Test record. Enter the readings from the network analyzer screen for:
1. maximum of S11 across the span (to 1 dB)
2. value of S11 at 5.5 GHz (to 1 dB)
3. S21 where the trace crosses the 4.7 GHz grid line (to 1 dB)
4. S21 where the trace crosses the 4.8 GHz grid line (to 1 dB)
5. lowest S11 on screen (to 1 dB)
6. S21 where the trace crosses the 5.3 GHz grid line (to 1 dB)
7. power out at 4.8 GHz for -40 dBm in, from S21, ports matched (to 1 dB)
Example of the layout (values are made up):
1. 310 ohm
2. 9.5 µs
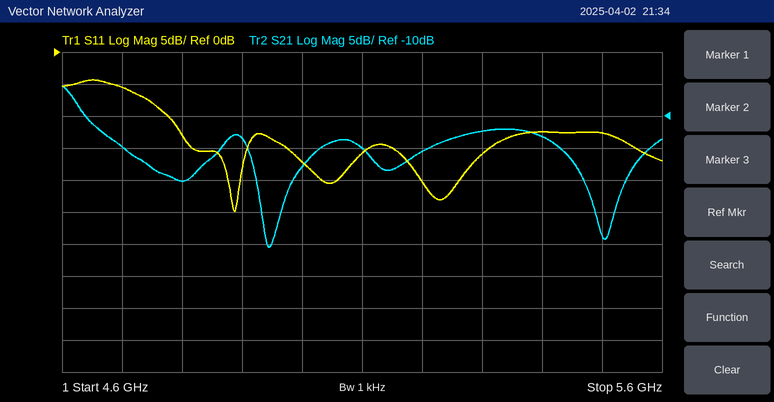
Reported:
1. -4 dB
2. -13 dB
3. -15 dB
4. -20 dB
5. -25 dB
6. -12 dB
7. -60 dBm
